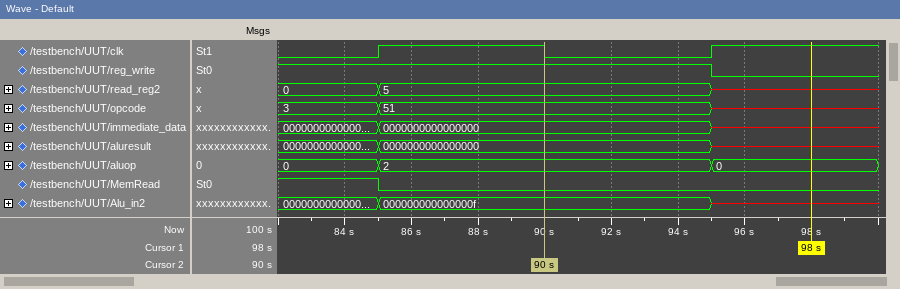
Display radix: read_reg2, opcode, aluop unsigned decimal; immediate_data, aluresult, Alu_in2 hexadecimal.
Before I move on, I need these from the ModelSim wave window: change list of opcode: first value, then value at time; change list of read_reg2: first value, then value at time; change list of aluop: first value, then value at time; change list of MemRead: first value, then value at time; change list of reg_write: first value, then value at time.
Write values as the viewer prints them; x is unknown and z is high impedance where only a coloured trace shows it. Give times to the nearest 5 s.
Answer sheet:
3, 51 at 85 s, x at 95 s
0, 5 at 85 s, x at 95 s
0, 2 at 85 s, 0 at 95 s
1, 0 at 85 s
1, 0 at 95 s
